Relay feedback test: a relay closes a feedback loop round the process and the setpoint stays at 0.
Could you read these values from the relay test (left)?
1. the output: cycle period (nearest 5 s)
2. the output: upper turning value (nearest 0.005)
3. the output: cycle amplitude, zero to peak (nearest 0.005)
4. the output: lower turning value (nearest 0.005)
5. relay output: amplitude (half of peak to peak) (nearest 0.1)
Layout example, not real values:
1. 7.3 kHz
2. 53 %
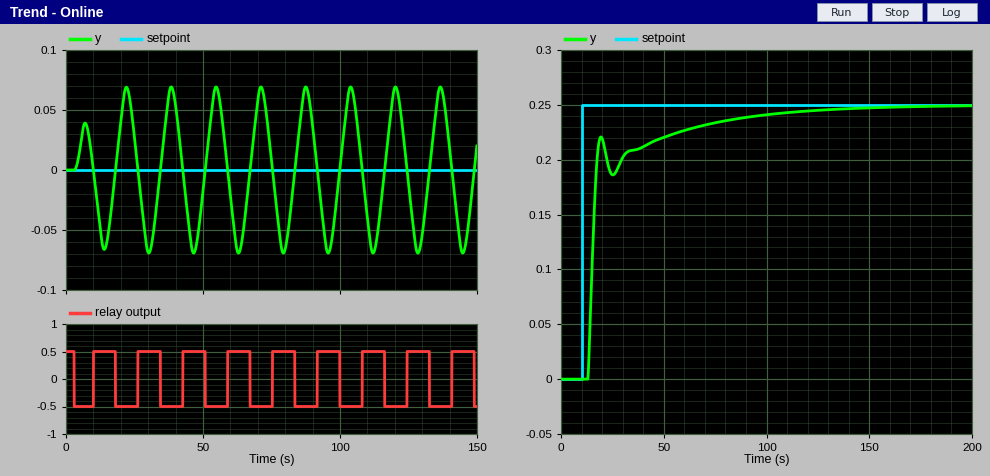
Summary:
1. 15 s
2. 0.070
3. 0.070
4. -0.070
5. 0.5
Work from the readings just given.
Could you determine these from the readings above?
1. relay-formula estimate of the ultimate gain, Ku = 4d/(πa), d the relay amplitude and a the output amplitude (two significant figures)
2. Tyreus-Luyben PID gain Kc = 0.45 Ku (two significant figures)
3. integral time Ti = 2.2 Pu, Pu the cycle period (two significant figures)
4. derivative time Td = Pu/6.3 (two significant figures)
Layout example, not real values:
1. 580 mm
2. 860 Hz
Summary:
1. 9.1
2. 4.1
3. 33 s
4. 2.4 s
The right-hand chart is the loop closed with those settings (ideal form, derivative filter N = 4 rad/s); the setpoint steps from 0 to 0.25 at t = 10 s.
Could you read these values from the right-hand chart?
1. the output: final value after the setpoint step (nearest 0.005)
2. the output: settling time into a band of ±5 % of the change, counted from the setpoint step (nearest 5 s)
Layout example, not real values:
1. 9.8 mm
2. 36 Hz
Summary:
1. 0.250
2. 75 s
